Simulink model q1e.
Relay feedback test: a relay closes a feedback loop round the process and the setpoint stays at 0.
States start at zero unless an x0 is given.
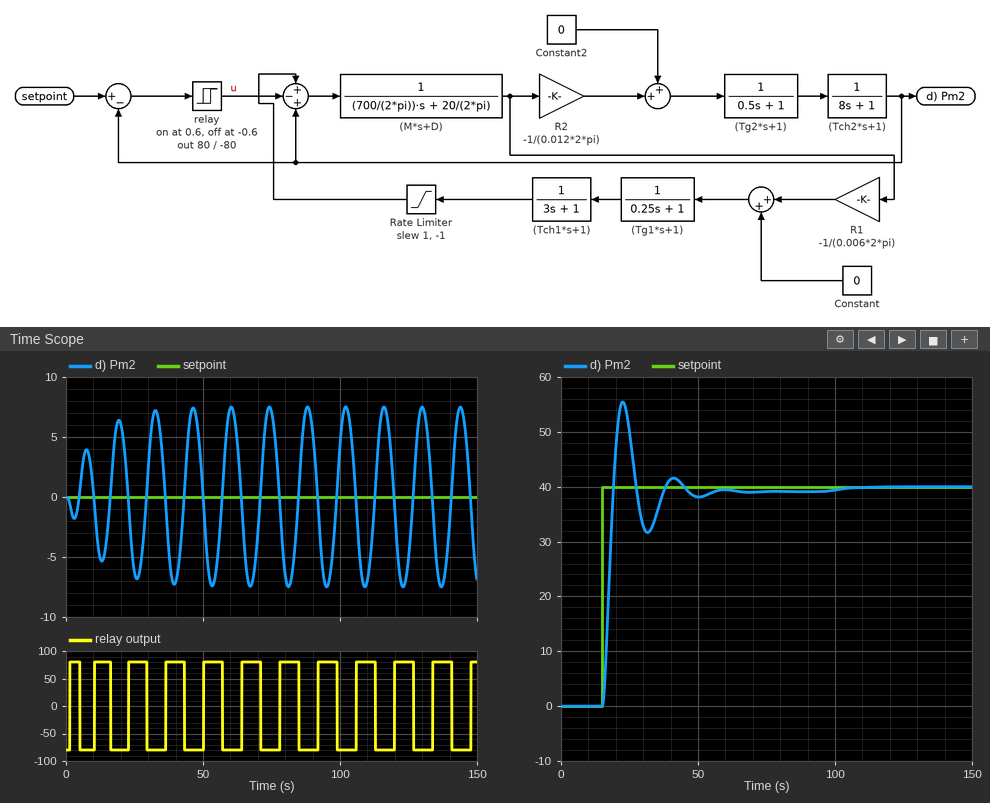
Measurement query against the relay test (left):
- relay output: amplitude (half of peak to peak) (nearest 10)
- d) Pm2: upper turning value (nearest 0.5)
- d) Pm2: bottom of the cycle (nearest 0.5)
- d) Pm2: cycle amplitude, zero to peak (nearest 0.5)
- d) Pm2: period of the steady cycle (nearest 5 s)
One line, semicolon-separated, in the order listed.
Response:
80; 7.5; -7.5; 7.5; 15 s
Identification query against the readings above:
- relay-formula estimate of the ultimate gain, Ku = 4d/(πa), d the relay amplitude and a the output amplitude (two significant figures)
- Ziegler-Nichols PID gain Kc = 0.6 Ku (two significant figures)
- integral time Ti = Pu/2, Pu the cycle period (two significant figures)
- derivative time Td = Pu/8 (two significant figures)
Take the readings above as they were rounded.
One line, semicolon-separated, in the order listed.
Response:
14; 8.4; 7.5 s; 1.9 s
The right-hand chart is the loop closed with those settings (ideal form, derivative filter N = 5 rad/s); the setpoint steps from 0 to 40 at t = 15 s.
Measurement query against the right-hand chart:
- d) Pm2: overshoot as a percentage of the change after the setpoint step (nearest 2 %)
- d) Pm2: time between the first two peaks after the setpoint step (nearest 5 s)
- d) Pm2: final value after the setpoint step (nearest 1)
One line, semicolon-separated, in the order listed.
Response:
38 %; 20 s; 40
